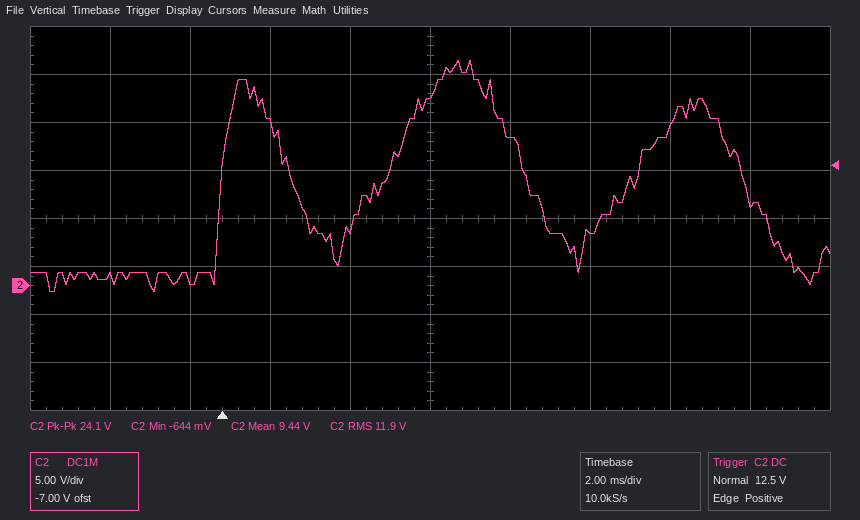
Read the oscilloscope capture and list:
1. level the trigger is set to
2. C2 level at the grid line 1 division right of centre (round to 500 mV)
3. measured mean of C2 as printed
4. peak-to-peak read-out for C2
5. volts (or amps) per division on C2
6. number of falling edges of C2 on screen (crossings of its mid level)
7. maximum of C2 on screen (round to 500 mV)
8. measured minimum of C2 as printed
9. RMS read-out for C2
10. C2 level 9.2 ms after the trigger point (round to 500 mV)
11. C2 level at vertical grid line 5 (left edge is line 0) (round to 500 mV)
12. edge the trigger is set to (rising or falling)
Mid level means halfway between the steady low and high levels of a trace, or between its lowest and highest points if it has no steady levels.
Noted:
12.5 V
15.5 V
9.44 V
24.1 V
5 V
3
23.5 V
-644 mV
11.9 V
5.5 V
20.0 V
rising
